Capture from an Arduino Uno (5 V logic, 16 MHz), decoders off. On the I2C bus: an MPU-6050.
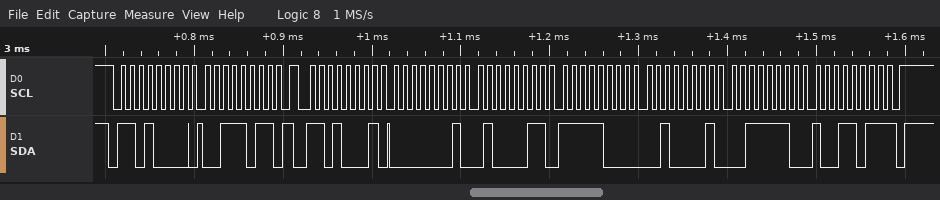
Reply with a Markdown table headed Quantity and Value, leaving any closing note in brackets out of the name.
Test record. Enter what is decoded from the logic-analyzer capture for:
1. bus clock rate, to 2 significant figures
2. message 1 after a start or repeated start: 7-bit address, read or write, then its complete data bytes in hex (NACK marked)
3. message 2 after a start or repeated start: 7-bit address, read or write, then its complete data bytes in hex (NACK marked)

| Quantity | Value |
|---|---|
| bus clock rate, to 2 significant figures | 100 kHz |
| message 1 after a start or repeated start: 7-bit address, read or write, then its complete data bytes in hex | 0x68 write: 3B |
| message 2 after a start or repeated start: 7-bit address, read or write, then its complete data bytes in hex | 0x68 read: 01 43 F8 21 3E 9B NACK |
